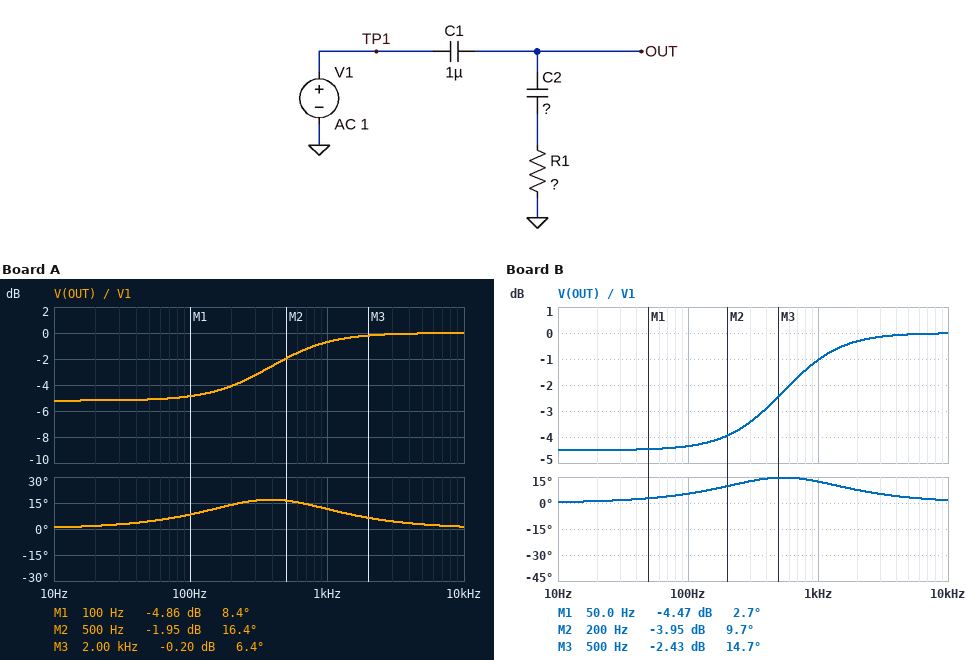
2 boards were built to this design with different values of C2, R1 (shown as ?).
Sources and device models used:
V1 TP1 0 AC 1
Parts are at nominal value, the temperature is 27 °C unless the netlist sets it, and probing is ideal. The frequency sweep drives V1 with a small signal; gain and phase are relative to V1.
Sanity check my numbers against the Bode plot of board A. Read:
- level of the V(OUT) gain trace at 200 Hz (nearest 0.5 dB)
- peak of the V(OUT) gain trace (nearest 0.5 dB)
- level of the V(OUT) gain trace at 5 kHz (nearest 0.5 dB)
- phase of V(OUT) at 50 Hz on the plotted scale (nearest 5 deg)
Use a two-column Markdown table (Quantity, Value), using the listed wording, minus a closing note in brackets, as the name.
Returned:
| Quantity | Value |
|---|---|
| level of the V(OUT) gain trace at 200 Hz | -4.0 dB |
| peak of the V(OUT) gain trace | 0 dB |
| level of the V(OUT) gain trace at 5 kHz | 0 dB |
| phase of V(OUT) at 50 Hz on the plotted scale | 5 deg |
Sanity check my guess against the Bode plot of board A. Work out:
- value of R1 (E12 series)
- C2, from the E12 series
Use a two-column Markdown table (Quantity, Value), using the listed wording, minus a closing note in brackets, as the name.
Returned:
| Quantity | Value |
|---|---|
| value of R1 | 680 Ω |
| C2, from the E12 series | 820 nF |
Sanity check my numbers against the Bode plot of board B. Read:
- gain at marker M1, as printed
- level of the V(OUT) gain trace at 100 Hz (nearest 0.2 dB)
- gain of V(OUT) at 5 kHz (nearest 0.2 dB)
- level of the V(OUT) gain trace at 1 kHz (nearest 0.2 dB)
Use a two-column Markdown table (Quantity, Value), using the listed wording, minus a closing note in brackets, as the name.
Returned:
| Quantity | Value |
|---|---|
| gain at marker M1, as printed | -4.47 dB |
| level of the V(OUT) gain trace at 100 Hz | -4.4 dB |
| gain of V(OUT) at 5 kHz | 0 dB |
| level of the V(OUT) gain trace at 1 kHz | -1.0 dB |
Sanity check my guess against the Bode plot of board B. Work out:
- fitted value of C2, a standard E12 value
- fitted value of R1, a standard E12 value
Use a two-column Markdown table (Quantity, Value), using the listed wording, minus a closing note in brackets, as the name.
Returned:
| Quantity | Value |
|---|---|
| fitted value of C2, a standard E12 value | 680 nF |
| fitted value of R1, a standard E12 value | 560 Ω |
